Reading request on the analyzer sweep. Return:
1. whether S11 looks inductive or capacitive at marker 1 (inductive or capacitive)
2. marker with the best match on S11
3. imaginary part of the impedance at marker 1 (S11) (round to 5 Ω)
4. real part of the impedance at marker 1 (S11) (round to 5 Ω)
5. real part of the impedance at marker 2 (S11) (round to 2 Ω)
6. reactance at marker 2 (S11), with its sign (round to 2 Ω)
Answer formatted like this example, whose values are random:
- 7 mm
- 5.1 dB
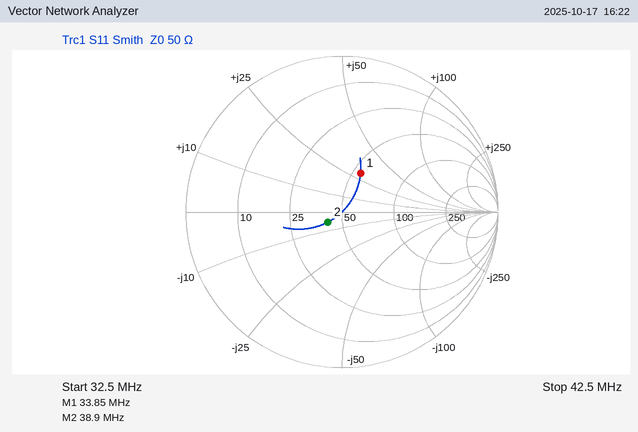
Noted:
- inductive
- marker 2
- +30 Ω
- 55 Ω
- 42 Ω
- -6 Ω
